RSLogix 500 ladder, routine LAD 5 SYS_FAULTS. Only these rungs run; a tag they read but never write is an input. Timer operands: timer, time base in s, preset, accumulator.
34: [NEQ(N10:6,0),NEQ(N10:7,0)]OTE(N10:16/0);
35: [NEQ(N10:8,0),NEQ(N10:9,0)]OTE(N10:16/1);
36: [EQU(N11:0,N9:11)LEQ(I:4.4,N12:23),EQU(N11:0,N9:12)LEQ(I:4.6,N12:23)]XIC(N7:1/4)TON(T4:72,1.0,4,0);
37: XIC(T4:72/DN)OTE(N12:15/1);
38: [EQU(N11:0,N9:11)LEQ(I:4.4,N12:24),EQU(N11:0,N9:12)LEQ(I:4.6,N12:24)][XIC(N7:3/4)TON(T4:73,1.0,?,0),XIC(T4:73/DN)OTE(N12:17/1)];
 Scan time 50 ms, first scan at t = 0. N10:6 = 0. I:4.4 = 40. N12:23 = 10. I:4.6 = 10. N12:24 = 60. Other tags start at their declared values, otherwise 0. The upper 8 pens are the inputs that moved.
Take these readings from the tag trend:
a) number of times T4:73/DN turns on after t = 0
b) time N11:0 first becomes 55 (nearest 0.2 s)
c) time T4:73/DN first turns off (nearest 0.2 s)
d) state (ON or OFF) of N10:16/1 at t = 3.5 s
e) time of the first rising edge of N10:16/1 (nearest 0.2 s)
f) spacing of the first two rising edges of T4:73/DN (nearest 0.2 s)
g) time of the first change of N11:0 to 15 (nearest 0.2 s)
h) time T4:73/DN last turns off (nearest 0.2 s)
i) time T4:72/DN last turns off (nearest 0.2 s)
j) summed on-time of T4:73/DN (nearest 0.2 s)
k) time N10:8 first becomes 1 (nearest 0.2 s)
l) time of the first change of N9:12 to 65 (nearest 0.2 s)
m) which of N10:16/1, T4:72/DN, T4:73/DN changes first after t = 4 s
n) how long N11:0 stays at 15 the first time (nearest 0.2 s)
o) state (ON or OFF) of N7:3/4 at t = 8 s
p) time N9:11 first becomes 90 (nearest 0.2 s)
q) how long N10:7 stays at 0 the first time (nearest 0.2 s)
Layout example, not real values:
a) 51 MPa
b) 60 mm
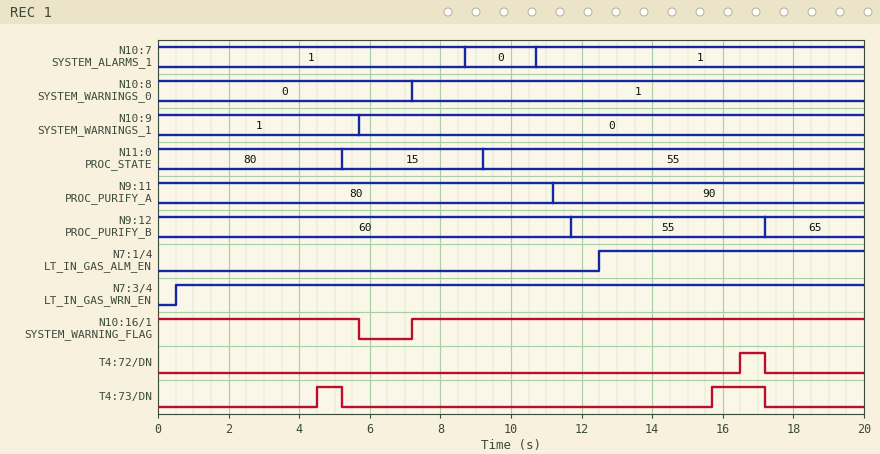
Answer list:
a) 2
b) 9.2 s
c) 5.2 s
d) ON
e) 7.2 s
f) 11.2 s
g) 5.2 s
h) 17.2 s
i) 17.2 s
j) 2.2 s
k) 7.2 s
l) 17.2 s
m) T4:73/DN
n) 4.0 s
o) ON
p) 11.2 s
q) 2.0 s
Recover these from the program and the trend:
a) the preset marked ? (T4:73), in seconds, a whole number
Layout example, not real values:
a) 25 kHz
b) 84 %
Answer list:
a) 4 s
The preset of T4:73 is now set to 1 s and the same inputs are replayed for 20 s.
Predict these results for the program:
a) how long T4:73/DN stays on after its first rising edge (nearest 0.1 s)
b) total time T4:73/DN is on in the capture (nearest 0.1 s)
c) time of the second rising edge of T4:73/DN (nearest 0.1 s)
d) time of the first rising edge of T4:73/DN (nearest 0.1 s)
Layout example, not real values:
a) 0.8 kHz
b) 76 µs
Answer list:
a) 3.7 s
b) 8.2 s
c) 12.7 s
d) 1.5 s
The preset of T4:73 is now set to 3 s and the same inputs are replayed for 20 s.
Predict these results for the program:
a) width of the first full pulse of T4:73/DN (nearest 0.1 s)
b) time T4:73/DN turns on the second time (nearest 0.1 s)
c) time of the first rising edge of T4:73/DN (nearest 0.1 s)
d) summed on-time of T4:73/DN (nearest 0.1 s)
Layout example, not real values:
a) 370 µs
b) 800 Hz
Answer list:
a) 1.7 s
b) 14.7 s
c) 3.5 s
d) 4.2 s
